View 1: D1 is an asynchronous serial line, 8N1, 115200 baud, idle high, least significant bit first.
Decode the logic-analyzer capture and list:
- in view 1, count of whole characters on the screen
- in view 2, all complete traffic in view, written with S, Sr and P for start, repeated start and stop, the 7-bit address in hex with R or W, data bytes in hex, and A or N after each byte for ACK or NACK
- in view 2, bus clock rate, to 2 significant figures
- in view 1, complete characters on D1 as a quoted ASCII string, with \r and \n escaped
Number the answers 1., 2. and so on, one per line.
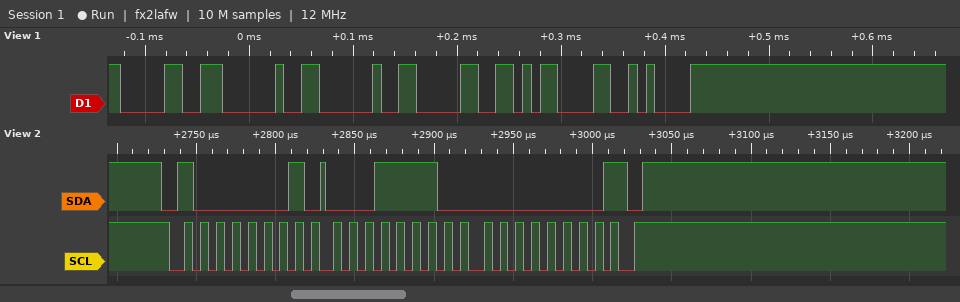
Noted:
1. 6
2. S 40R A 1E A 00 N P
3. 100 kHz
4. "0  0\r\n"
